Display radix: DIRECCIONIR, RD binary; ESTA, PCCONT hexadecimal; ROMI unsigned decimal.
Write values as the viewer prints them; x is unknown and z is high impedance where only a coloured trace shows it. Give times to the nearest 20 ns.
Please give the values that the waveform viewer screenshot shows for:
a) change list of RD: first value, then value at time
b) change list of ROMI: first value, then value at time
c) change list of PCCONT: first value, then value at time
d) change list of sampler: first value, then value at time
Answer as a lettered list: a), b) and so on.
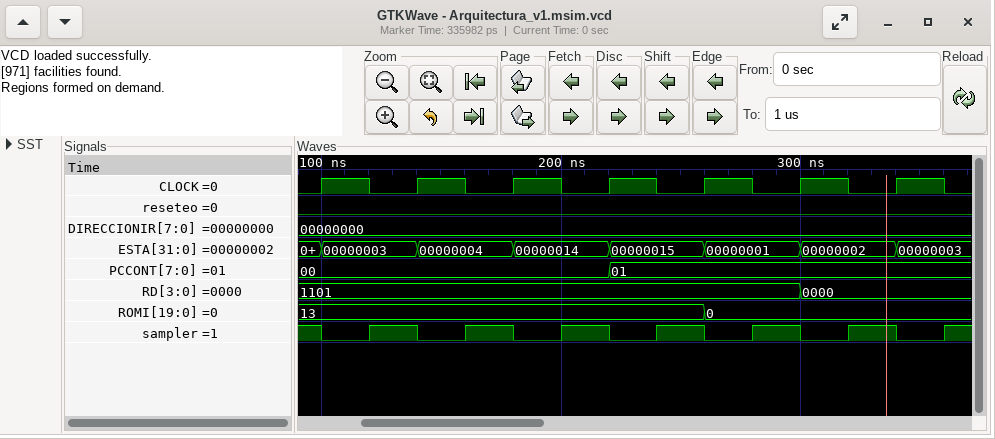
a) 1101, 0000 at 300 ns
b) 13, 0 at 260 ns
c) 00, 01 at 220 ns
d) 1, 0 at 100 ns, 1 at 120 ns, 0 at 140 ns, 1 at 160 ns, 0 at 180 ns, 1 at 200 ns, 0 at 220 ns, 1 at 240 ns, 0 at 260 ns, 1 at 280 ns, 0 at 300 ns, 1 at 320 ns, 0 at 340 ns, 1 at 360 ns
